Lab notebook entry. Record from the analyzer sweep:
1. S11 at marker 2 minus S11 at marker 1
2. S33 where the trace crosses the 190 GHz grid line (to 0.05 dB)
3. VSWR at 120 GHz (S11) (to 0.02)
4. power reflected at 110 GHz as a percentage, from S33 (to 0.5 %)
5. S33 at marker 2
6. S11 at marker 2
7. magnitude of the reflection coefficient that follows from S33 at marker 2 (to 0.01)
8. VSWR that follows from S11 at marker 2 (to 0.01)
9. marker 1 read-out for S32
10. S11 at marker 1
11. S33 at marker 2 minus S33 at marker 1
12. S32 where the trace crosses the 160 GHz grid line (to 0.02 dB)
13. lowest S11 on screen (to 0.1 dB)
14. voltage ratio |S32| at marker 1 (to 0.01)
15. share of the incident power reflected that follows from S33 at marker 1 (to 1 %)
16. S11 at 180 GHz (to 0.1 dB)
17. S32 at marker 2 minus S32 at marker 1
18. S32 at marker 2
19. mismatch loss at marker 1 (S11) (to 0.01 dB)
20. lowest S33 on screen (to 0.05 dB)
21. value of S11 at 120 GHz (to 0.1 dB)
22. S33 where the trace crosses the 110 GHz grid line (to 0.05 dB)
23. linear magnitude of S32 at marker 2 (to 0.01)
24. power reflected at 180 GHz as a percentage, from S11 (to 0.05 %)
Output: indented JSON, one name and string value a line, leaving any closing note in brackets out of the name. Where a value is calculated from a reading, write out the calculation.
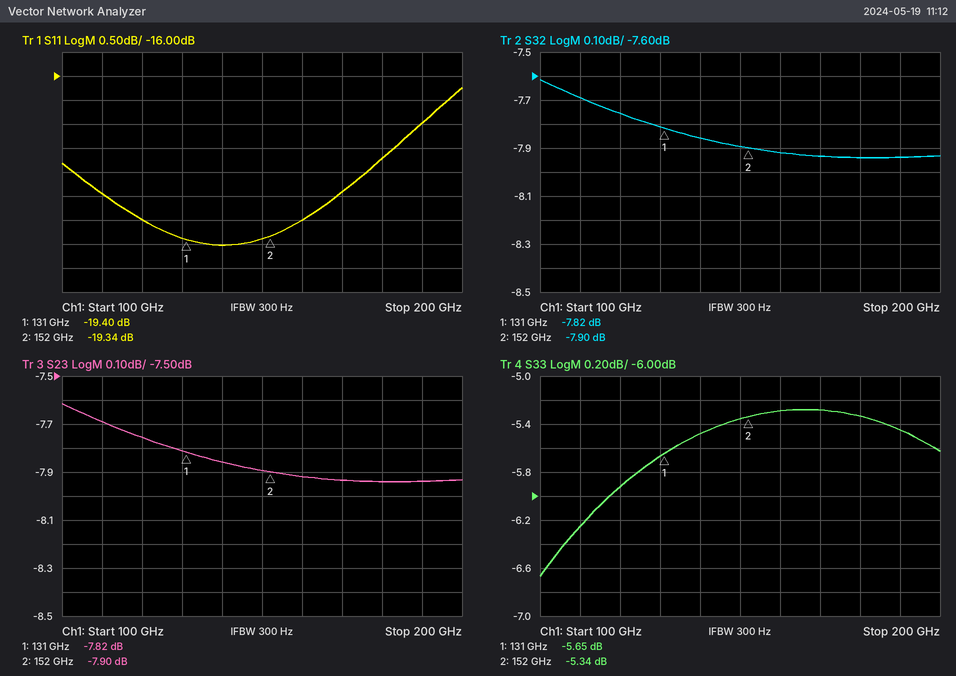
{
  "S11 at marker 2 minus S11 at marker 1": "-19.34 − (-19.4) = 0.06 dB",
  "S33 where the trace crosses the 190 GHz grid line": "-5.45 dB",
  "VSWR at 120 GHz (S11)": "|Γ| = 10^(-19/20) = 0.1122; VSWR = (1 + 0.1122)/(1 − 0.1122) ≈ 1.25, so 1.26 to the nearest 0.02",
  "power reflected at 110 GHz as a percentage, from S33": "10^(-6.25/10) ≈ 23.7 %, so 23.5 % to the nearest 0.5 %",
  "S33 at marker 2": "-5.34 dB",
  "S11 at marker 2": "-19.34 dB",
  "magnitude of the reflection coefficient that follows from S33 at marker 2": "10^(-5.34/20) ≈ 0.54",
  "VSWR that follows from S11 at marker 2": "(1 + 0.1079)/(1 − 0.1079) ≈ 1.24",
  "marker 1 read-out for S32": "-7.82 dB",
  "S11 at marker 1": "-19.40 dB",
  "S33 at marker 2 minus S33 at marker 1": "-5.34 − (-5.65) = 0.31 dB",
  "S32 where the trace crosses the 160 GHz grid line": "-7.92 dB",
  "lowest S11 on screen": "-19.5 dB",
  "voltage ratio |S32| at marker 1": "10^(-7.82/20) ≈ 0.41",
  "share of the incident power reflected that follows from S33 at marker 1": "10^(-5.65/10) ≈ 27 %",
  "S11 at 180 GHz": "-17.7 dB",
  "S32 at marker 2 minus S32 at marker 1": "-7.9 − (-7.82) = -0.08 dB",
  "S32 at marker 2": "-7.90 dB",
  "mismatch loss at marker 1 (S11)": "−10 log10(1 − 10^(-19.4/10)) ≈ 0.05 dB",
  "lowest S33 on screen": "-6.65 dB",
  "value of S11 at 120 GHz": "-19.0 dB",
  "S33 where the trace crosses the 110 GHz grid line": "-6.25 dB",
  "linear magnitude of S32 at marker 2": "10^(-7.9/20) ≈ 0.40",
  "power reflected at 180 GHz as a percentage, from S11": "10^(-17.7/10) ≈ 1.70 %"
}
